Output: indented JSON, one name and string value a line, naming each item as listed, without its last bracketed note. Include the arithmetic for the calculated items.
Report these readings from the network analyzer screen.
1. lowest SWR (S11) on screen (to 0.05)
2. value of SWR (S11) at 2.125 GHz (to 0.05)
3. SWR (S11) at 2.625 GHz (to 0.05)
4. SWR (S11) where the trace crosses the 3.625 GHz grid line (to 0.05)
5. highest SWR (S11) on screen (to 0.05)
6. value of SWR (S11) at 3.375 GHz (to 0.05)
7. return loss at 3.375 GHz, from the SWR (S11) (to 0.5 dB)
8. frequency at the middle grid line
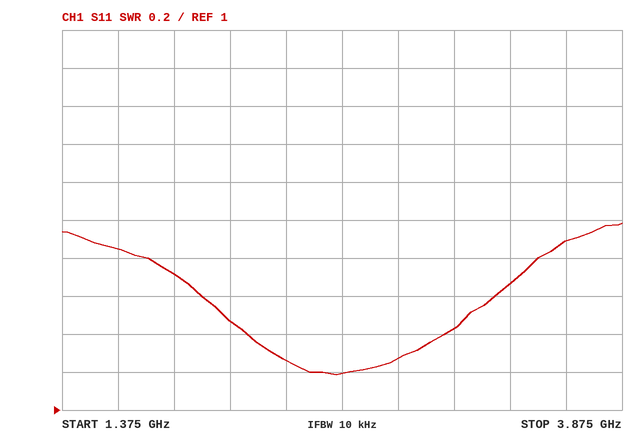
{
  "lowest SWR (S11) on screen": "1.20",
  "value of SWR (S11) at 2.125 GHz": "1.45",
  "SWR (S11) at 2.625 GHz": "1.20",
  "SWR (S11) where the trace crosses the 3.625 GHz grid line": "1.90",
  "highest SWR (S11) on screen": "2.00",
  "value of SWR (S11) at 3.375 GHz": "1.65",
  "return loss at 3.375 GHz, from the SWR (S11)": "−20 log10((1.65 − 1)/(1.65 + 1)) ≈ 12.2 dB, so 12.0 dB to the nearest 0.5 dB",
  "frequency at the middle grid line": "2.625 GHz"
}
